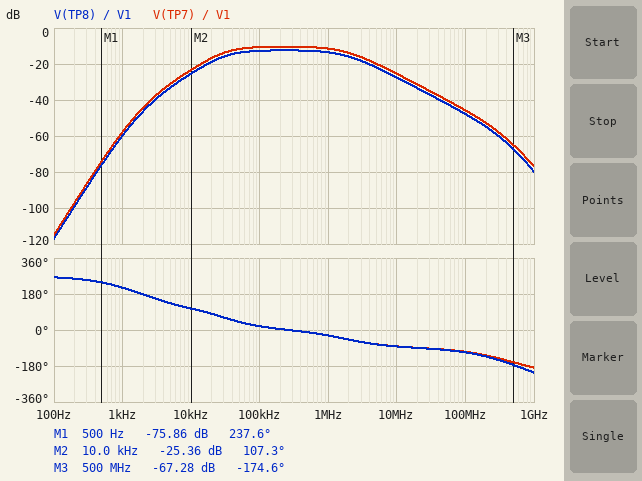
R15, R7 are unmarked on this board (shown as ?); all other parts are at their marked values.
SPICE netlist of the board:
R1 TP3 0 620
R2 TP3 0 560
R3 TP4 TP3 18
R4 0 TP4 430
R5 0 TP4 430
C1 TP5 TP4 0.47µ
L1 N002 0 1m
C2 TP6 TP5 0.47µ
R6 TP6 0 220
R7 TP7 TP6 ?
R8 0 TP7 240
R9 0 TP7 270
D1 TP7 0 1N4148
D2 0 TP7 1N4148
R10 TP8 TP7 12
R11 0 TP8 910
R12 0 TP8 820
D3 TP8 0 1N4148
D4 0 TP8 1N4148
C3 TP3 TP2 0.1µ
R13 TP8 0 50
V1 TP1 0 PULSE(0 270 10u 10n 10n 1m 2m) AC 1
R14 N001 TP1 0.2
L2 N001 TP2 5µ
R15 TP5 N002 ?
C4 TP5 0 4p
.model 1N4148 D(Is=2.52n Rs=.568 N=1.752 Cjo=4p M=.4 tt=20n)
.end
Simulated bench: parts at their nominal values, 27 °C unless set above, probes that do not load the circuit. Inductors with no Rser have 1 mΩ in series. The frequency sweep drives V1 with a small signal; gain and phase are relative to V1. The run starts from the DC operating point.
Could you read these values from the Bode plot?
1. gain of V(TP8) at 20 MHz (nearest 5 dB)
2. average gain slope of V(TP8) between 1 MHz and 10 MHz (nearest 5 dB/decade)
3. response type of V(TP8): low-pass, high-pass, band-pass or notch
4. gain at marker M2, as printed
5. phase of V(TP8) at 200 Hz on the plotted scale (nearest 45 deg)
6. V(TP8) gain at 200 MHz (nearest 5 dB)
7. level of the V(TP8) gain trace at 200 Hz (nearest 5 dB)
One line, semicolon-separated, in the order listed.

-35 dB; -15 dB/decade; band-pass; -25.36 dB; 270 deg; -55 dB; -100 dB
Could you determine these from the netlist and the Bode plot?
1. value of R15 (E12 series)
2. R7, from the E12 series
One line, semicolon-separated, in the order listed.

100 Ω; 56 Ω
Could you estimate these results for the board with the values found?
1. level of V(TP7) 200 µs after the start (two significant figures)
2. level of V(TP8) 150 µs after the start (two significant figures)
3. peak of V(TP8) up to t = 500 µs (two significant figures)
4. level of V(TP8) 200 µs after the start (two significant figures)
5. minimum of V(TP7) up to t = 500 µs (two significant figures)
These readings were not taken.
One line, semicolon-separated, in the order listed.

120 mV; -52 mV; 870 mV; 94 mV; -970 mV
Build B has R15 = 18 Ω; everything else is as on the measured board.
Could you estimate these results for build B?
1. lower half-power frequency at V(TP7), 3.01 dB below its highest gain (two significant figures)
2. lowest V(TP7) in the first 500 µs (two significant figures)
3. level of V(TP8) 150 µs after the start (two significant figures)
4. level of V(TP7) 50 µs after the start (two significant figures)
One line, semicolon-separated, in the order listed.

29 kHz; -1.1 V; 330 mV; -870 mV
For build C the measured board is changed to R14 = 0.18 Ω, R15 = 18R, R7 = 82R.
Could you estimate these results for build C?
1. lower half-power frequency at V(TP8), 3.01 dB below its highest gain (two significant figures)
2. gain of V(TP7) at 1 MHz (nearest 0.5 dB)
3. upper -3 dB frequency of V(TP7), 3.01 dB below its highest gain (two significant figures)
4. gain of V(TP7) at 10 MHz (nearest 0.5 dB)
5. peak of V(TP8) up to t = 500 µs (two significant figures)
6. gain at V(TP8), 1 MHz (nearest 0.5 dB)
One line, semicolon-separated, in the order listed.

26 kHz; -13.0 dB; 1.9 MHz; -26.5 dB; 840 mV; -15.0 dB
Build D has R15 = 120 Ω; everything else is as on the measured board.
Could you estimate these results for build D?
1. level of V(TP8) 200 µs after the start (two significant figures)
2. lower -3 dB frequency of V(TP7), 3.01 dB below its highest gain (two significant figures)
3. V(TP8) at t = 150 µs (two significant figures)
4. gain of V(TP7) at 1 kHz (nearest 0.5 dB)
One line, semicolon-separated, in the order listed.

66 mV; 33 kHz; -110 mV; -56.5 dB
